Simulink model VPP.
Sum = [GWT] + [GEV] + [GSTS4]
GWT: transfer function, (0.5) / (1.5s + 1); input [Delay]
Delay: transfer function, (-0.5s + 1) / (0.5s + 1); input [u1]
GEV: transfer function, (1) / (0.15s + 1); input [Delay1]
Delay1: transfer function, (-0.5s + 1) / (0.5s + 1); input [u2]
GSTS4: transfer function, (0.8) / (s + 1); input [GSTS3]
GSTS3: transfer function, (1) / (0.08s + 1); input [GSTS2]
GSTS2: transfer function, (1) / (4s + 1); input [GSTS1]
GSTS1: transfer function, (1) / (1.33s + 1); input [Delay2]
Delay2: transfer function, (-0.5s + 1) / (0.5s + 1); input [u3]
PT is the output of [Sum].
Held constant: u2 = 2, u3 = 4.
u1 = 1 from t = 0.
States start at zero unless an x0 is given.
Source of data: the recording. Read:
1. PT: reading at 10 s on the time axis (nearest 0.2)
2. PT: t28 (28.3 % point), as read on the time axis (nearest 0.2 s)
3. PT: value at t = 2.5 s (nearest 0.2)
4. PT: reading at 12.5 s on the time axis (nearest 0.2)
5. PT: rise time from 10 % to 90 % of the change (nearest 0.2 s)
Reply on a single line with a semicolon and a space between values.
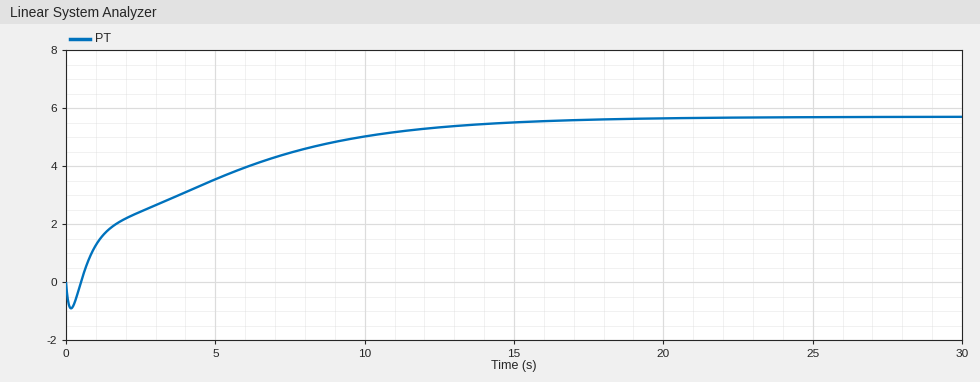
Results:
5.0; 1.2 s; 2.4; 5.4; 10.0 s
